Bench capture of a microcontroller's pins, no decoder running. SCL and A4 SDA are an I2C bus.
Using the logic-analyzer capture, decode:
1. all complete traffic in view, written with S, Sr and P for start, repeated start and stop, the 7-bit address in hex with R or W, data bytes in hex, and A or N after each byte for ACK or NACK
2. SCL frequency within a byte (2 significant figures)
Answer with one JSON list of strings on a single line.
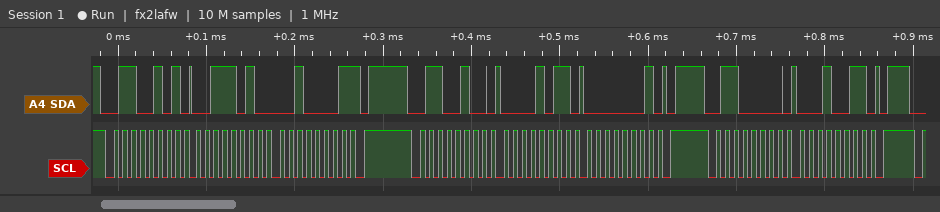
["S 32R A 3A A 21 N P S 32W A 0B A 01 A P S 30W A 13 A P", "100 kHz"]
